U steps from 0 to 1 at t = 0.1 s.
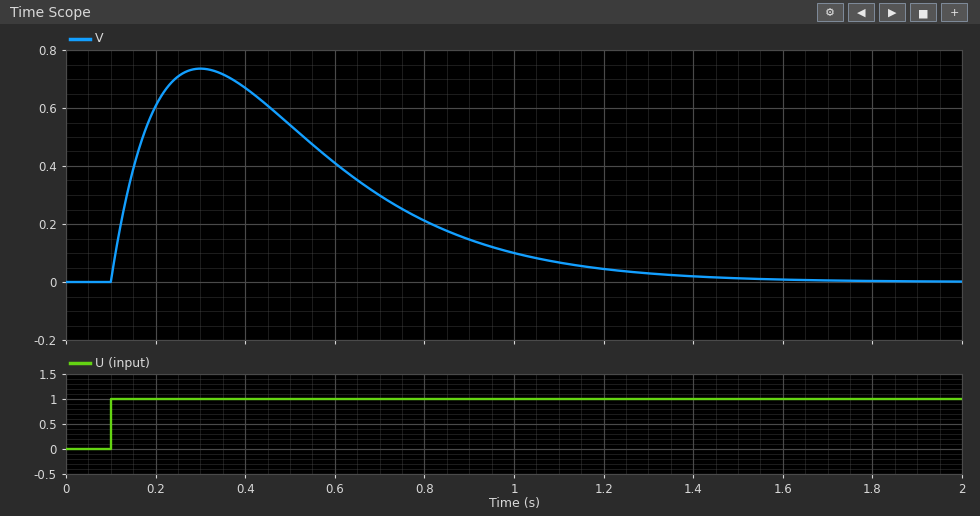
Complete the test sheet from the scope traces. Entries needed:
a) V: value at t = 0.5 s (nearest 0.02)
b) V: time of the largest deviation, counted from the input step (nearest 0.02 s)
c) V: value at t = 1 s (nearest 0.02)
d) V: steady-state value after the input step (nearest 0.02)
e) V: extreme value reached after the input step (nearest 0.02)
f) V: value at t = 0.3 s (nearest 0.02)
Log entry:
0.54
0.20 s
0.10
0.00
0.74
0.74
